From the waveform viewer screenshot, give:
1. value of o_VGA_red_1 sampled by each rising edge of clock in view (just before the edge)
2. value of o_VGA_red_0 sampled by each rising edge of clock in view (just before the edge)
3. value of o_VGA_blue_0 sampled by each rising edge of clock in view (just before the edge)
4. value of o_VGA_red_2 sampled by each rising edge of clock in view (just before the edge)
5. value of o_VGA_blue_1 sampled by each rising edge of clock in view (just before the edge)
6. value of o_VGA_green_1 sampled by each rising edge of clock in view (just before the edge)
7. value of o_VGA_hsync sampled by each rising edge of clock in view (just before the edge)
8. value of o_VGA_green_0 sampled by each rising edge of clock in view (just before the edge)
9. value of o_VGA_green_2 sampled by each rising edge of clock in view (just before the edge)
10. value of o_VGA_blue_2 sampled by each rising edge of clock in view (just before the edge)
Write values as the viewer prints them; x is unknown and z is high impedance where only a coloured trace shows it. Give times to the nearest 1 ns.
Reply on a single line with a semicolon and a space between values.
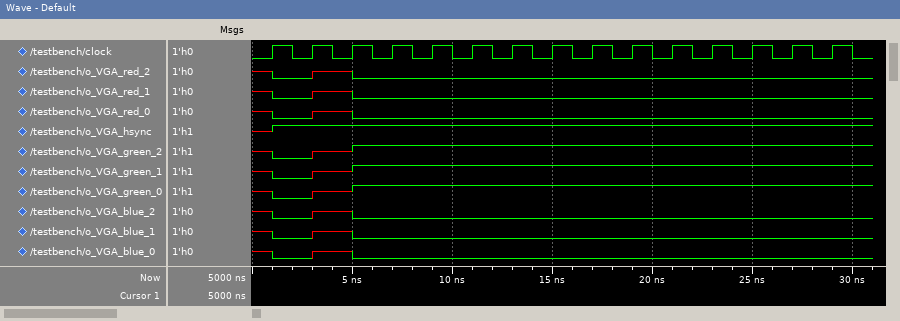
x 0 x 0 0 0 0 0 0 0 0 0 0 0 0; x 0 x 0 0 0 0 0 0 0 0 0 0 0 0; x 0 x 0 0 0 0 0 0 0 0 0 0 0 0; x 0 x 0 0 0 0 0 0 0 0 0 0 0 0; x 0 x 0 0 0 0 0 0 0 0 0 0 0 0; x 0 x 1 1 1 1 1 1 1 1 1 1 1 1; x 1 1 1 1 1 1 1 1 1 1 1 1 1 1; x 0 x 1 1 1 1 1 1 1 1 1 1 1 1; x 0 x 1 1 1 1 1 1 1 1 1 1 1 1; x 0 x 0 0 0 0 0 0 0 0 0 0 0 0
